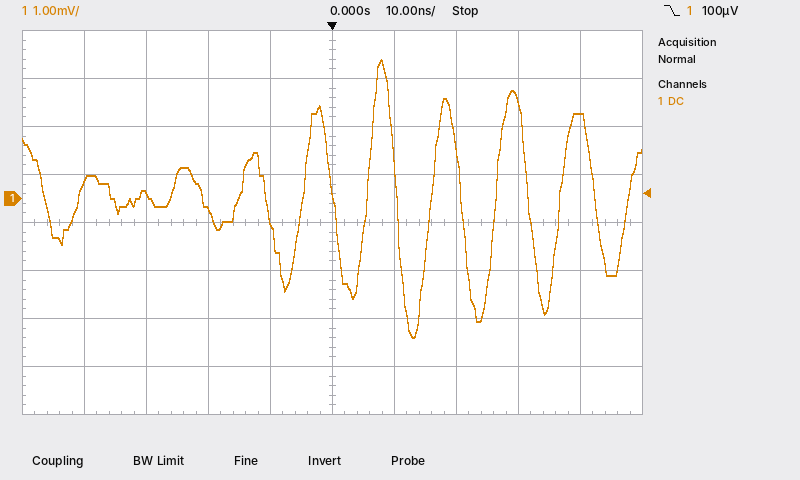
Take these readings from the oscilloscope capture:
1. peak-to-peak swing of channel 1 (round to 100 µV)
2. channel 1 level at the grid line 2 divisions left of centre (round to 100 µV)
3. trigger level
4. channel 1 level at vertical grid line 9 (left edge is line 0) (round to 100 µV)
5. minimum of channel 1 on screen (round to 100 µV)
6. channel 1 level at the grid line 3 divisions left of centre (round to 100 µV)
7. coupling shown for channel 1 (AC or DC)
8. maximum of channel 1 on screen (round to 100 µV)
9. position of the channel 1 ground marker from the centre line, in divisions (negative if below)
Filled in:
5.8 mV
-200 µV
100 µV
1.8 mV
-2.9 mV
100 µV
DC
2.9 mV
+0.5 div
